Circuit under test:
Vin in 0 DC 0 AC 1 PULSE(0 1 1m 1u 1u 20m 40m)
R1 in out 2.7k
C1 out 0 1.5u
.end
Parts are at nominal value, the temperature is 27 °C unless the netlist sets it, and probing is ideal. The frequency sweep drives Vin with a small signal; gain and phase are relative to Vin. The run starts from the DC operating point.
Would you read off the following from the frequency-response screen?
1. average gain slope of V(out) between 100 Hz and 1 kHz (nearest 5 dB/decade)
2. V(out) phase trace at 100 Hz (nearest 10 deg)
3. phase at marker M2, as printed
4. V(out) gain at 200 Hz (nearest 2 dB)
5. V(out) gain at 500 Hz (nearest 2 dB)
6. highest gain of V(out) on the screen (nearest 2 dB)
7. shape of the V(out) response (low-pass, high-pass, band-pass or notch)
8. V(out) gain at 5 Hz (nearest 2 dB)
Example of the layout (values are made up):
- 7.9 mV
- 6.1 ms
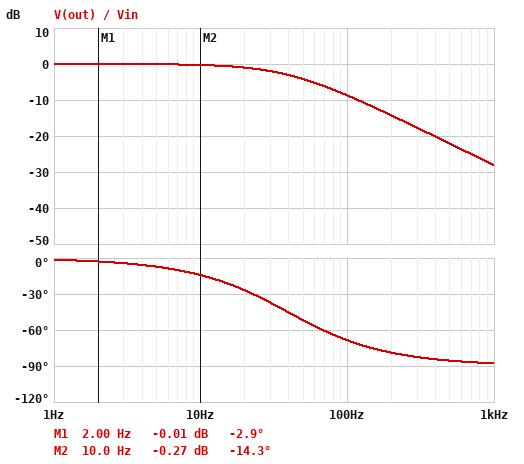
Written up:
- -20 dB/decade
- -70 deg
- -14.3 deg
- -14 dB
- -22 dB
- 0 dB
- low-pass
- 0 dB
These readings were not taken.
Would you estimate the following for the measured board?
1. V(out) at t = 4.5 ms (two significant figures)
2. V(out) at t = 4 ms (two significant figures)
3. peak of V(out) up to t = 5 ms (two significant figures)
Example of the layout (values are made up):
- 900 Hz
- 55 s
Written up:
- 580 mV
- 520 mV
- 630 mV
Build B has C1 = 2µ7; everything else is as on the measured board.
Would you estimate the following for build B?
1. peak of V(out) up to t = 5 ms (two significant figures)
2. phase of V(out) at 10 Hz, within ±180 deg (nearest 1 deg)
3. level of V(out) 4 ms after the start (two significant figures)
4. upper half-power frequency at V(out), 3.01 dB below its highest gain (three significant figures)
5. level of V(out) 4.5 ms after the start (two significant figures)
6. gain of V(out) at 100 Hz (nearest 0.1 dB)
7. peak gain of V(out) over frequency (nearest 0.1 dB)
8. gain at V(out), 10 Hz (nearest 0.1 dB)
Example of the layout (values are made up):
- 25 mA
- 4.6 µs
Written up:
- 420 mV
- -25 deg
- 340 mV
- 21.8 Hz
- 380 mV
- -13.4 dB
- 0 dB
- -0.8 dB
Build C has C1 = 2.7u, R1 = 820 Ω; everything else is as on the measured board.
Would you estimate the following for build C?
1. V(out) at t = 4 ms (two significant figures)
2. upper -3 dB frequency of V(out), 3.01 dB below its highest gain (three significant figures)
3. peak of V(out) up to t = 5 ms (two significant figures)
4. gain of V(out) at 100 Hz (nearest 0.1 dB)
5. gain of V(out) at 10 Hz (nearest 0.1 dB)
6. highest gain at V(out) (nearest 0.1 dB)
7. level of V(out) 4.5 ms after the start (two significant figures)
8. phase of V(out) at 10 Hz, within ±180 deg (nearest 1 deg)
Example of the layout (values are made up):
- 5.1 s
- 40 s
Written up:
- 740 mV
- 71.9 Hz
- 840 mV
- -4.7 dB
- -0.1 dB
- 0 dB
- 790 mV
- -8 deg
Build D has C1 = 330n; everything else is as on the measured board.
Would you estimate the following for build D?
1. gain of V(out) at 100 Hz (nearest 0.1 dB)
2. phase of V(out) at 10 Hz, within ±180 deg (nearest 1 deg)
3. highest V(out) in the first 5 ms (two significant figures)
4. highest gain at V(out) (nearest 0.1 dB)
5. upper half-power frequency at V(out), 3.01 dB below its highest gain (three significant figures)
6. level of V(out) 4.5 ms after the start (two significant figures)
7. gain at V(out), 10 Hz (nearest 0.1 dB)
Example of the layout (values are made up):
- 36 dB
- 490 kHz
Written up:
- -1.2 dB
- -3 deg
- 990 mV
- 0 dB
- 179 Hz
- 980 mV
- 0 dB
